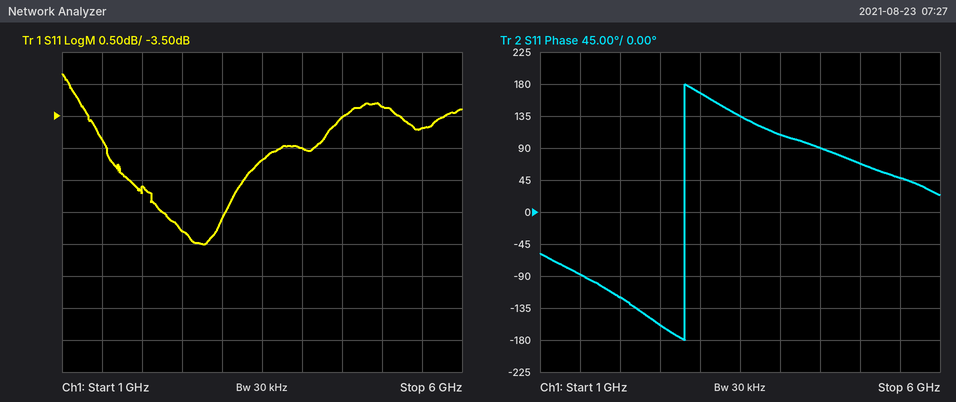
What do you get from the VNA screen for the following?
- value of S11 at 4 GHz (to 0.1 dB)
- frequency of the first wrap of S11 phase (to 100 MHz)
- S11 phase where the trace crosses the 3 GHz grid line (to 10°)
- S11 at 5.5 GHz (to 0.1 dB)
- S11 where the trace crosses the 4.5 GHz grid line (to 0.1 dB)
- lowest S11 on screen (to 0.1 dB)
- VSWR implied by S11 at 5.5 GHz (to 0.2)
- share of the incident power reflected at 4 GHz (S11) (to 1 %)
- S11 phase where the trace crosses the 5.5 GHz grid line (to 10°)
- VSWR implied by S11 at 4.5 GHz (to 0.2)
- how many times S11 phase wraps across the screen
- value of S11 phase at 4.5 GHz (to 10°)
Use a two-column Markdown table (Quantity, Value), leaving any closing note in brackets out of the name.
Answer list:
| Quantity | Value |
|---|---|
| value of S11 at 4 GHz | -4.0 dB |
| frequency of the first wrap of S11 phase | 2.8 GHz |
| S11 phase where the trace crosses the 3 GHz grid line | 170° |
| S11 at 5.5 GHz | -3.7 dB |
| S11 where the trace crosses the 4.5 GHz grid line | -3.5 dB |
| lowest S11 on screen | -5.5 dB |
| VSWR implied by S11 at 5.5 GHz | 4.8 |
| share of the incident power reflected at 4 GHz (S11) | 40 % |
| S11 phase where the trace crosses the 5.5 GHz grid line | 50° |
| VSWR implied by S11 at 4.5 GHz | 5.0 |
| how many times S11 phase wraps across the screen | 1 |
| value of S11 phase at 4.5 GHz | 90° |
